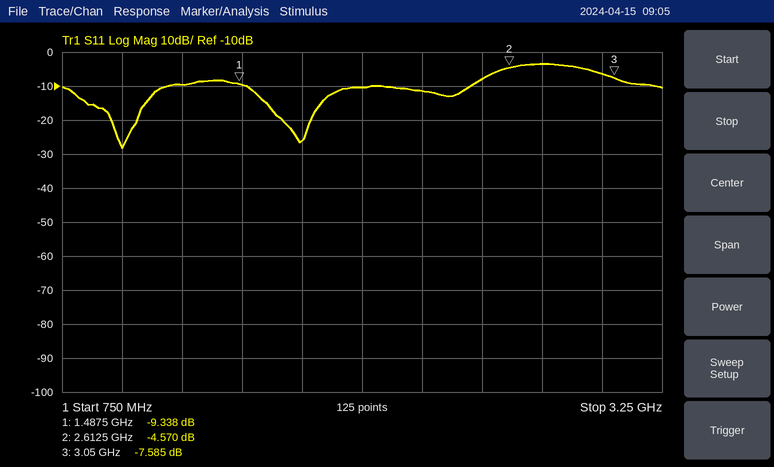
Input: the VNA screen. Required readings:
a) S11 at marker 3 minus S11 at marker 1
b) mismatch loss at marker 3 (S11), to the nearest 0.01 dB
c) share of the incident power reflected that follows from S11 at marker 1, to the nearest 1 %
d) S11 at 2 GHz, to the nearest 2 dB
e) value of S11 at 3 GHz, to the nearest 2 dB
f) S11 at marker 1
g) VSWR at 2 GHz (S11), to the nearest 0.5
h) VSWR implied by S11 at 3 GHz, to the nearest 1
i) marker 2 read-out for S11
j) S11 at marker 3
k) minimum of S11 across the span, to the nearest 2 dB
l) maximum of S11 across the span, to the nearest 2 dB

1.753 dB
0.83 dB
12 %
-10 dB
-6 dB
-9.338 dB
2.0
3
-4.570 dB
-7.585 dB
-28 dB
-4 dB
